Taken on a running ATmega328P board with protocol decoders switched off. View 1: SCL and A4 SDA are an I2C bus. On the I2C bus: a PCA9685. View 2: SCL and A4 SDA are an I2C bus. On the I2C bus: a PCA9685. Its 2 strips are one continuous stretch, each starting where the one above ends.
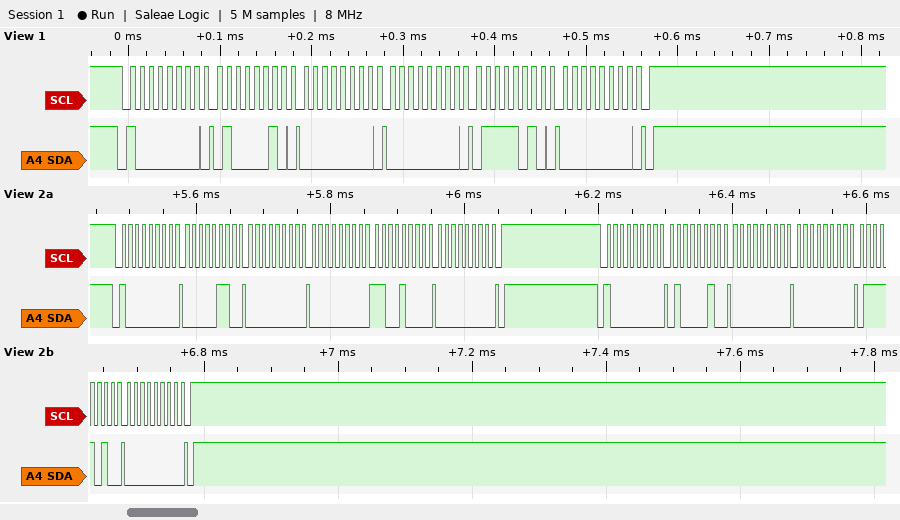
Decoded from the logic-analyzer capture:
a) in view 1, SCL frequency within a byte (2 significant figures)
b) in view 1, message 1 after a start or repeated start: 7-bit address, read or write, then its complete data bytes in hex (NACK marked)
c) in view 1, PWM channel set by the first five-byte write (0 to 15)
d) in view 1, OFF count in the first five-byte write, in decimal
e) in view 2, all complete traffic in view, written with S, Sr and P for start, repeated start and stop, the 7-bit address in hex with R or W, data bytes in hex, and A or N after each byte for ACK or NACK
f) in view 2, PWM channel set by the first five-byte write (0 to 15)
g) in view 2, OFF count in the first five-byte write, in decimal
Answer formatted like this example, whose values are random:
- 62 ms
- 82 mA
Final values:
- 100 kHz
- 0x40 write: 42 00 00 7A 00
- 15
- 122
- S 40W A 06 A 00 A 00 A C8 A 00 A P S 40W A 42 A 00 A 00 A 7A A 00 A P
- 0
- 200
